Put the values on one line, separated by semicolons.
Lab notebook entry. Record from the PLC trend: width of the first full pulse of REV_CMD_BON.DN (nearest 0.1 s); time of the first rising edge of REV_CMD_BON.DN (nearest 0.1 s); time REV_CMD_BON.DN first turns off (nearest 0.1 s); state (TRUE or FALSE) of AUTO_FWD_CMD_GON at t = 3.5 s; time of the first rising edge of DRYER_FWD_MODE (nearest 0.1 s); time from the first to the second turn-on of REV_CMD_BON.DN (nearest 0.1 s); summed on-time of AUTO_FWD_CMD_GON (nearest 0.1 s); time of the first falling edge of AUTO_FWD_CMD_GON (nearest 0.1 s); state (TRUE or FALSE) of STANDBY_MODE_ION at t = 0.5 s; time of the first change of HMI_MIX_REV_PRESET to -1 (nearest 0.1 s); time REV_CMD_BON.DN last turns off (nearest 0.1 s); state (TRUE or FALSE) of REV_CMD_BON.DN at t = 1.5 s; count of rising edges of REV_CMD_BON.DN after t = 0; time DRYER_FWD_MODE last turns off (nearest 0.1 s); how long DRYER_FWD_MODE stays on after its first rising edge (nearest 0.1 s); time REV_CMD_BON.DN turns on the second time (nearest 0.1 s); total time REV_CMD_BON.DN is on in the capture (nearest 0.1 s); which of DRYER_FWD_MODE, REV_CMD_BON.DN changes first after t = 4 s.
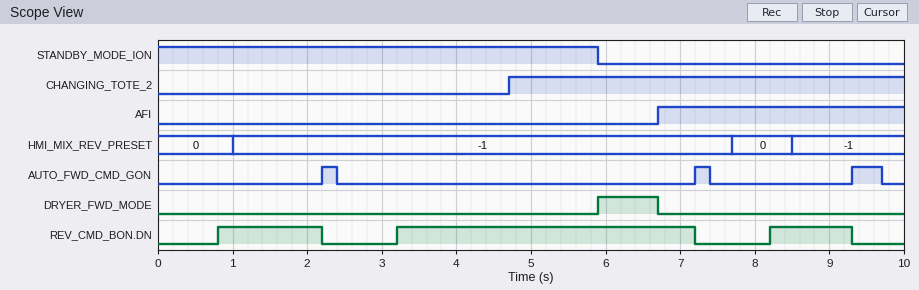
1.4 s; 0.8 s; 2.2 s; FALSE; 5.9 s; 2.4 s; 0.8 s; 2.4 s; TRUE; 1.0 s; 9.3 s; TRUE; 3; 6.7 s; 0.8 s; 3.2 s; 6.5 s; DRYER_FWD_MODE
